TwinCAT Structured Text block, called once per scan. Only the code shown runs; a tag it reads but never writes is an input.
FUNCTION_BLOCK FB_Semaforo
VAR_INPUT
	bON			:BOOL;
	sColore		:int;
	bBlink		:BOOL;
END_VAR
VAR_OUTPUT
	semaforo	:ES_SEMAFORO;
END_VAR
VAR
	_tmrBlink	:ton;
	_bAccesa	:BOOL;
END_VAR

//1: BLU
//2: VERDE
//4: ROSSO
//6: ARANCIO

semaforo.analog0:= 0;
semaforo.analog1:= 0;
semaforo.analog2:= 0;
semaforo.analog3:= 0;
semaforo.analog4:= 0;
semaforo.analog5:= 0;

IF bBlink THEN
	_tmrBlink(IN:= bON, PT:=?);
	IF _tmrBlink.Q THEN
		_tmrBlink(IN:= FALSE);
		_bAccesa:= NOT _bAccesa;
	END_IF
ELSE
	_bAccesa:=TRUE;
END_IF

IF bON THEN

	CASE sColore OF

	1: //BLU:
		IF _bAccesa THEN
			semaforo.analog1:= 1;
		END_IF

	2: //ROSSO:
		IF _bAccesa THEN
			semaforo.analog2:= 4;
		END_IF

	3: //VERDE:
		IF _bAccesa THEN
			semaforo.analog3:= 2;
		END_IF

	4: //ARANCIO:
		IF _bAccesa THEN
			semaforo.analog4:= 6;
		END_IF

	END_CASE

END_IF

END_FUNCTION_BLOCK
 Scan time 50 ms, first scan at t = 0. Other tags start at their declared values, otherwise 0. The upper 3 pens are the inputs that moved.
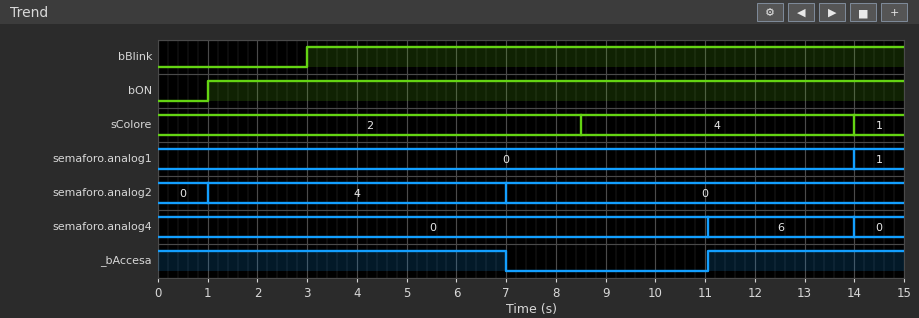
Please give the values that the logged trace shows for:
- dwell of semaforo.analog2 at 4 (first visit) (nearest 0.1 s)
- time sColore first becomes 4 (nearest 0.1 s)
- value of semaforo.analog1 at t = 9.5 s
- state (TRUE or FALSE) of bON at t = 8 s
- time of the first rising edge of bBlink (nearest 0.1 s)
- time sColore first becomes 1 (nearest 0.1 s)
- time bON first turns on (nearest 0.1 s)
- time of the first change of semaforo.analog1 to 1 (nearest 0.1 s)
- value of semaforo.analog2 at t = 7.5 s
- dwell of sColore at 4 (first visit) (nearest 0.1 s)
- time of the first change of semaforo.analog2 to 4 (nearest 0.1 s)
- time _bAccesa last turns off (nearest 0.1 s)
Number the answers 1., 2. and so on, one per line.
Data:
1. 6.0 s
2. 8.5 s
3. 0
4. TRUE
5. 3.0 s
6. 14.0 s
7. 1.0 s
8. 14.0 s
9. 0
10. 5.5 s
11. 1.0 s
12. 7.0 s
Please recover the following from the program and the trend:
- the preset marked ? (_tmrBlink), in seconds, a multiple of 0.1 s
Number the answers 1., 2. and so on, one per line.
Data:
1. 4.0 s
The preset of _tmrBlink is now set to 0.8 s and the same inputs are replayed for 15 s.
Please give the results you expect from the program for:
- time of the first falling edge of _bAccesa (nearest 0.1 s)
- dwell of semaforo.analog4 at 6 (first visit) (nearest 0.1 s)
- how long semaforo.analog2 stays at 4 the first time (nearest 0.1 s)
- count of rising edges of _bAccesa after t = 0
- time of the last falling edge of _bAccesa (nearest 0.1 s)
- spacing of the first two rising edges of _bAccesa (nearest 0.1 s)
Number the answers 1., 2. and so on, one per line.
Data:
1. 3.8 s
2. 0.4 s
3. 2.8 s
4. 7
5. 14.0 s
6. 1.7 s
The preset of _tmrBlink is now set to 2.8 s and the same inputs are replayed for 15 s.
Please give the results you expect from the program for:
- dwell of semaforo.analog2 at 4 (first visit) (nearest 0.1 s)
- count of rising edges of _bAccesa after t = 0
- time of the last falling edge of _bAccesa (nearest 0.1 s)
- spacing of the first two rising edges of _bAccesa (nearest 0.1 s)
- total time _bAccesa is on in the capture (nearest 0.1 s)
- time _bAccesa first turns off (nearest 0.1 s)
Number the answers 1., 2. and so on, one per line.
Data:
1. 4.8 s
2. 2
3. 11.5 s
4. 5.7 s
5. 9.3 s
6. 5.8 s
